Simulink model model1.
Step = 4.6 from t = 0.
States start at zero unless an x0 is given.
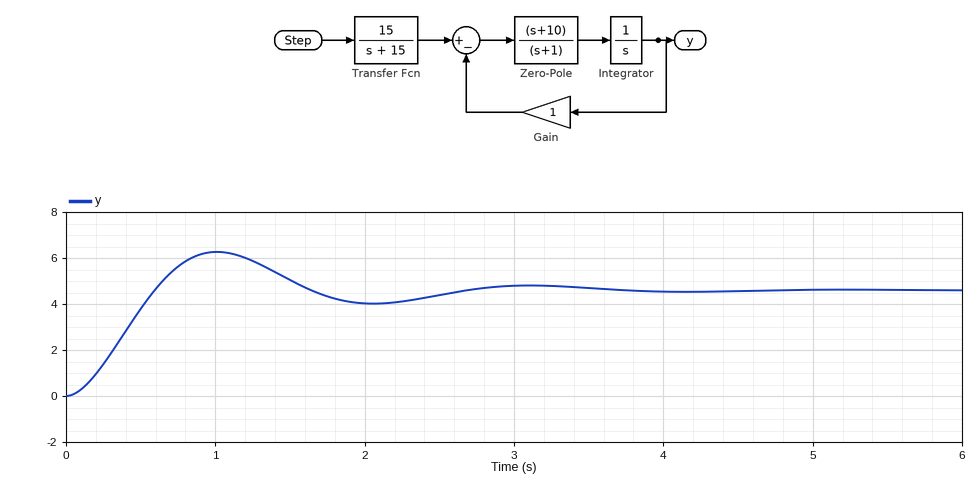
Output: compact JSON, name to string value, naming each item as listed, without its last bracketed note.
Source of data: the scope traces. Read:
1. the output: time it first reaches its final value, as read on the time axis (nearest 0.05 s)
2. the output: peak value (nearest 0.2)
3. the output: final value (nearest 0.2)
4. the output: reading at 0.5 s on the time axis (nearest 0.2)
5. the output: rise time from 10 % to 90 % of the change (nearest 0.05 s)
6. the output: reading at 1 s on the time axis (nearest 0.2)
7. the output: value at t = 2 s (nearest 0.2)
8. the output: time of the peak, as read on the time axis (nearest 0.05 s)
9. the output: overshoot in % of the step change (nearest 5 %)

{"the output: time it first reaches its final value, as read on the time axis": "0.60 s", "the output: peak value": "6.2", "the output: final value": "4.6", "the output: reading at 0.5 s on the time axis": "3.8", "the output: rise time from 10 % to 90 % of the change": "0.40 s", "the output: reading at 1 s on the time axis": "6.2", "the output: value at t = 2 s": "4.0", "the output: time of the peak, as read on the time axis": "1.00 s", "the output: overshoot in % of the step change": "35 %"}
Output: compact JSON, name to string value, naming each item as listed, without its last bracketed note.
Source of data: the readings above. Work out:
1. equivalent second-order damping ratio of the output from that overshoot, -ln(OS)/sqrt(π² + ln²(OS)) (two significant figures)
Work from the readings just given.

{"equivalent second-order damping ratio of the output from that overshoot, -ln(OS)/sqrt(π² + ln²(OS))": "0.32"}
